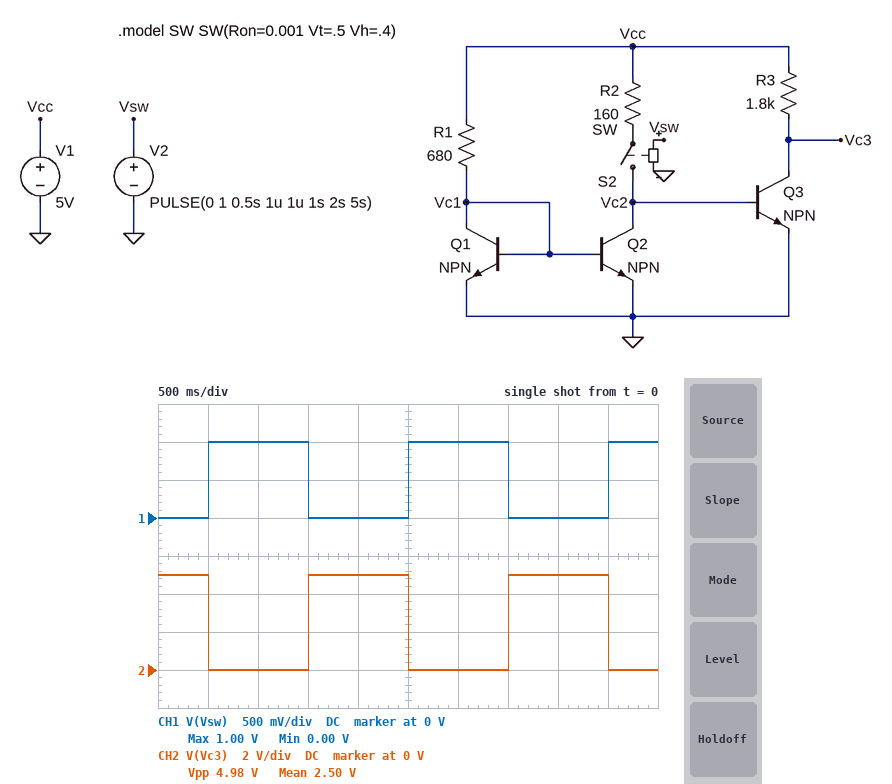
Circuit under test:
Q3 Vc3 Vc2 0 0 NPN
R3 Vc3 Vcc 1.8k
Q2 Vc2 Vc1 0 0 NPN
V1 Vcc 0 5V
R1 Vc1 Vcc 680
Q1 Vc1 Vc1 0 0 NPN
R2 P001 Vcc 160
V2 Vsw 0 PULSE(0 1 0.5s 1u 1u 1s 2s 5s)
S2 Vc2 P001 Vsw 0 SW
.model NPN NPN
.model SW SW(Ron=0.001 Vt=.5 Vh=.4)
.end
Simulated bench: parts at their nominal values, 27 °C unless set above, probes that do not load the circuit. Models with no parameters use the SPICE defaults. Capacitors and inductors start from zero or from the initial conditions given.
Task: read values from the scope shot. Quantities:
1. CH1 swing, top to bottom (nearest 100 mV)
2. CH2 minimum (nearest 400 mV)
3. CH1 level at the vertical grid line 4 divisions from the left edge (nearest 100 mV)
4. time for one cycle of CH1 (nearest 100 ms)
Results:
1.0 V
0 V
0 V
2.0 s
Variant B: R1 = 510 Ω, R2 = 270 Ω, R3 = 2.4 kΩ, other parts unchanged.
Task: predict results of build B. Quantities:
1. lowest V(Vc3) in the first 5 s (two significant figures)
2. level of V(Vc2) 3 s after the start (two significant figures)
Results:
21 mV
850 mV
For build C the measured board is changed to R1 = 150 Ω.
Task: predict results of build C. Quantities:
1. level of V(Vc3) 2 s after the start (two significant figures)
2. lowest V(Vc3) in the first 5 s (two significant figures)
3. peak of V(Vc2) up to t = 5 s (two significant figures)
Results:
5.0 V
5.0 V
670 mV
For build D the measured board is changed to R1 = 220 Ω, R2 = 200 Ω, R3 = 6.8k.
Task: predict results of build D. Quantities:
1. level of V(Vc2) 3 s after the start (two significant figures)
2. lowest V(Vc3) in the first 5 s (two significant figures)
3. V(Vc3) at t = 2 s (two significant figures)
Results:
820 mV
22 mV
5.0 V
